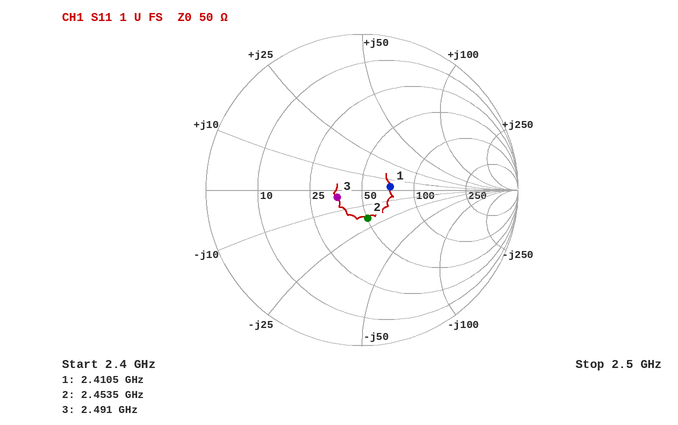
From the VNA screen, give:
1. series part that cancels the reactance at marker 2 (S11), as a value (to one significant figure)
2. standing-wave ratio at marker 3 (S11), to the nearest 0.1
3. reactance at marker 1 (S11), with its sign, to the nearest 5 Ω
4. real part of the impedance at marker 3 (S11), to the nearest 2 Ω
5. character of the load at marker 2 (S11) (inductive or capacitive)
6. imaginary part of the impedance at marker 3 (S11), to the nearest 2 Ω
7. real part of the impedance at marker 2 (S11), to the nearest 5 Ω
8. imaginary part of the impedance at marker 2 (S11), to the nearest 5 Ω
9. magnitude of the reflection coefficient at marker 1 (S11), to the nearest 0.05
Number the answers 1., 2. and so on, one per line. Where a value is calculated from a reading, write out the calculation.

1. L = 20 Ω/(2π × 2.4535 GHz) ≈ 1 nH
2. 1.4
3. +5 Ω
4. 36 Ω
5. capacitive
6. -4 Ω
7. 50 Ω
8. -20 Ω
9. 0.20
